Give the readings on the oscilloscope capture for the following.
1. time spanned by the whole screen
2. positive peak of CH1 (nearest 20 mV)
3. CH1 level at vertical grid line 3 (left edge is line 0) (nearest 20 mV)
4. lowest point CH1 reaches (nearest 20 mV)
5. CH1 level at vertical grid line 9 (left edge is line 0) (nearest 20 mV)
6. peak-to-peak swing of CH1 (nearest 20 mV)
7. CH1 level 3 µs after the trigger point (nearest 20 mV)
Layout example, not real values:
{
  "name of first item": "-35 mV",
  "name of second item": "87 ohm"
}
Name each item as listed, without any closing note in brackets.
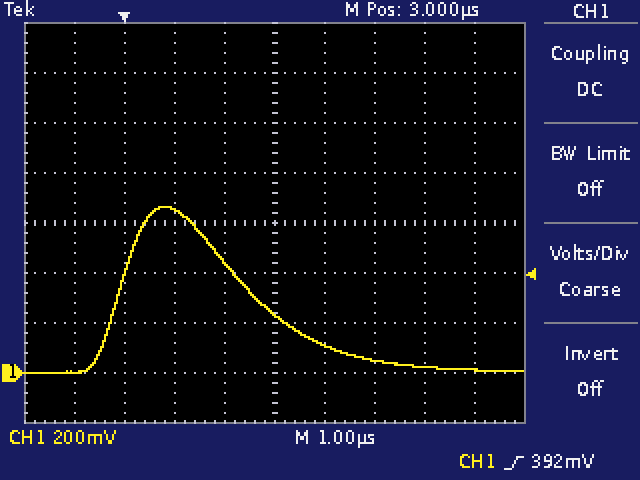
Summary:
{
  "time spanned by the whole screen": "10 µs",
  "positive peak of CH1": "660 mV",
  "CH1 level at vertical grid line 3 (left edge is line 0)": "660 mV",
  "lowest point CH1 reaches": "0 mV",
  "CH1 level at vertical grid line 9 (left edge is line 0)": "20 mV",
  "peak-to-peak swing of CH1": "660 mV",
  "CH1 level 3 µs after the trigger point": "240 mV"
}
